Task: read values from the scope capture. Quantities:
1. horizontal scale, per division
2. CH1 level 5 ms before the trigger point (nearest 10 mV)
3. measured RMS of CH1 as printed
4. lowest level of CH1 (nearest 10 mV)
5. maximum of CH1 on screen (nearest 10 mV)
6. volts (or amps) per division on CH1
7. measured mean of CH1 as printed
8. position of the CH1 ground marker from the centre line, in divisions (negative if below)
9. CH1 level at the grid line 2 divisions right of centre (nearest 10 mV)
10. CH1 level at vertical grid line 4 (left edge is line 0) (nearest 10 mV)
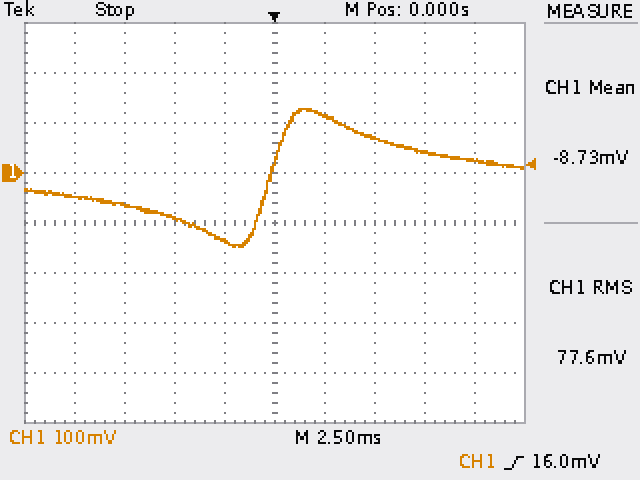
2.5 ms
-90 mV
77.6 mV
-150 mV
130 mV
100 mV
-8.73 mV
+1.0 div
70 mV
-140 mV
